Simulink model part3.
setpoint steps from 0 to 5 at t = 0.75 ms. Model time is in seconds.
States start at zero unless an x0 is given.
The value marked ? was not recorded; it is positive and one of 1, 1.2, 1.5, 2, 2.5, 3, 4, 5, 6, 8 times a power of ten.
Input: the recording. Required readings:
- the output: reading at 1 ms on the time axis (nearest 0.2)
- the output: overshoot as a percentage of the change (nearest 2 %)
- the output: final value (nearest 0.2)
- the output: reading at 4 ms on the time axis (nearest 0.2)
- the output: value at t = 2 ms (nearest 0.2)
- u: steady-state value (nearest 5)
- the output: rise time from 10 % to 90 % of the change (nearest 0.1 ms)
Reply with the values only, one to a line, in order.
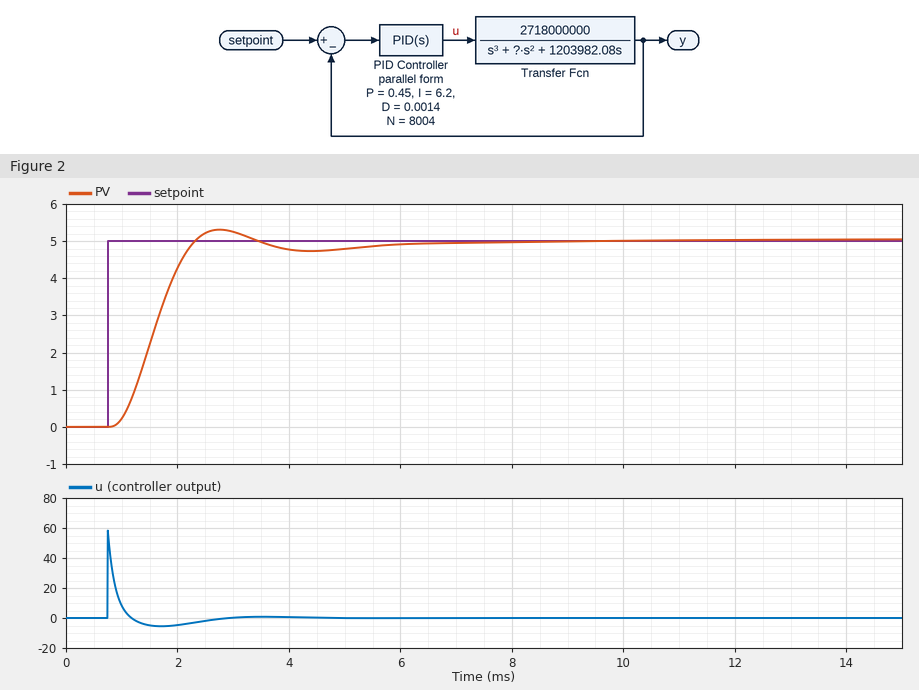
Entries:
0.2
6 %
5.0
4.8
4.2
0
1.0 ms
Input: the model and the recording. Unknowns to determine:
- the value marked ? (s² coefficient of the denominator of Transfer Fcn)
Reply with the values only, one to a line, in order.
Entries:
3000
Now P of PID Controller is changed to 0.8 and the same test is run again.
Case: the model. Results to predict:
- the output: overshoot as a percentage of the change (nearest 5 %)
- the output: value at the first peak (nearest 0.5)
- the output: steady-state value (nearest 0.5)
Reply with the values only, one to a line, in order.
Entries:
20 %
6.0
5.0
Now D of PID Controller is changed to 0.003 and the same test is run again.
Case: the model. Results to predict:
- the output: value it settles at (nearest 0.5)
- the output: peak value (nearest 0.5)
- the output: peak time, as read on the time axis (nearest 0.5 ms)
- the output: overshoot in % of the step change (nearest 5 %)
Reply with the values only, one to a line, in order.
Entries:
5.0
6.0
2.0 ms
25 %
